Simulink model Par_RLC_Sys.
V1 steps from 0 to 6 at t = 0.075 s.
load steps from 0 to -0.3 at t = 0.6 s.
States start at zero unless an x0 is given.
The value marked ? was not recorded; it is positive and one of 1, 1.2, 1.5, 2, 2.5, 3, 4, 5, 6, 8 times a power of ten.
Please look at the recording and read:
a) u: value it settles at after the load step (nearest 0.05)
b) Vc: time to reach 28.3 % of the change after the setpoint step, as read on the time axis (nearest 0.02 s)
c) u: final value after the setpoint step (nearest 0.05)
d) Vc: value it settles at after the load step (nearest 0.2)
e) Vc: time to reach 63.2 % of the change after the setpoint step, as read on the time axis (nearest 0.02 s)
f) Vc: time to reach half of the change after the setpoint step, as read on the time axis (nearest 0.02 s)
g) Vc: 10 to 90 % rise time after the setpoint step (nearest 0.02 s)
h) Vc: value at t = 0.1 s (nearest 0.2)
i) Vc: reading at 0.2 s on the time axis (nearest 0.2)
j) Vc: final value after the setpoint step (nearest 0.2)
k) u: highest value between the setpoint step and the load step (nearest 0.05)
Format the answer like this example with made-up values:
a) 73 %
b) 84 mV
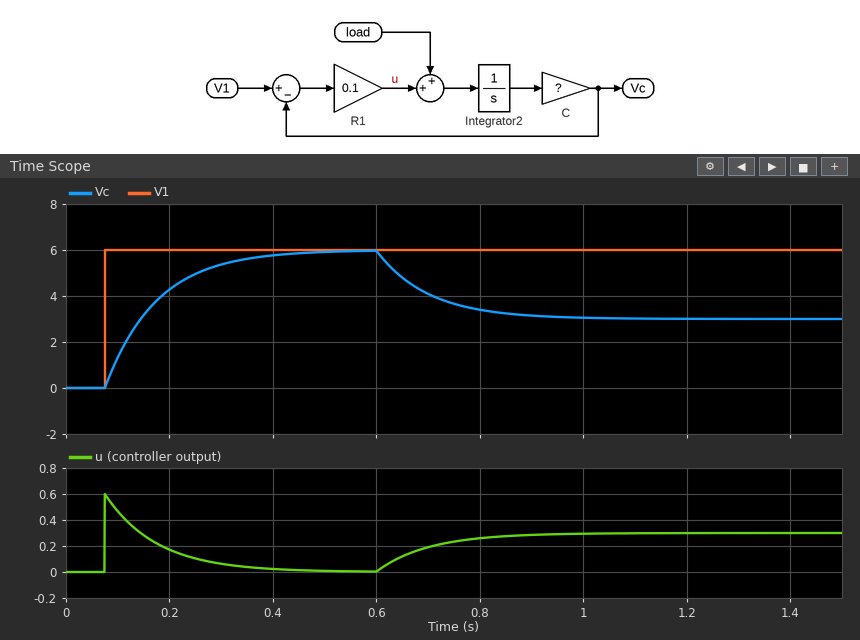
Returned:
a) 0.30
b) 0.10 s
c) 0.00
d) 3.0
e) 0.18 s
f) 0.14 s
g) 0.22 s
h) 1.4
i) 4.2
j) 6.0
k) 0.60
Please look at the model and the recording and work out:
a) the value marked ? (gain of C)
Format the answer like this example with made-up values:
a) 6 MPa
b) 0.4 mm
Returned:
a) 100
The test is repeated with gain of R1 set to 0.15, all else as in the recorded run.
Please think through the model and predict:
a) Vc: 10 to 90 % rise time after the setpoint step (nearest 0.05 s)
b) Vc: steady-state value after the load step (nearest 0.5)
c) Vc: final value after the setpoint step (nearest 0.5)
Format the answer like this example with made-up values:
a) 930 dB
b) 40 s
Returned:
a) 0.15 s
b) 4.0
c) 6.0
